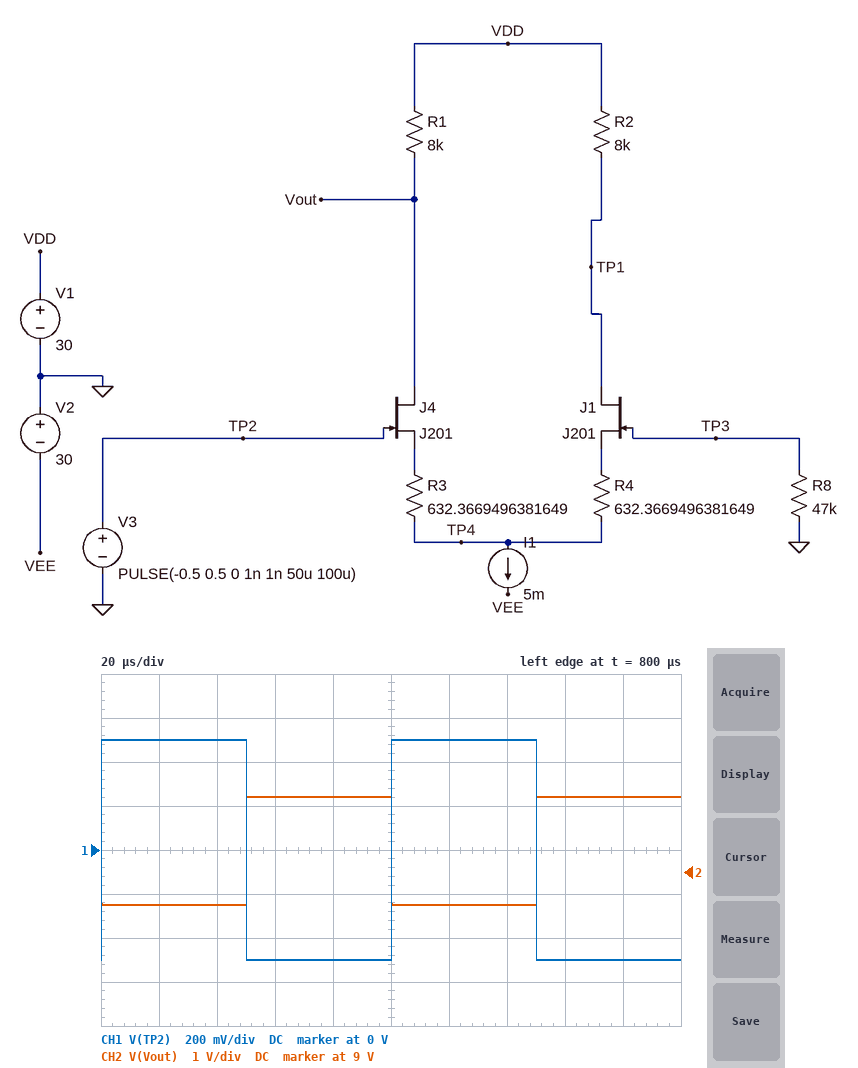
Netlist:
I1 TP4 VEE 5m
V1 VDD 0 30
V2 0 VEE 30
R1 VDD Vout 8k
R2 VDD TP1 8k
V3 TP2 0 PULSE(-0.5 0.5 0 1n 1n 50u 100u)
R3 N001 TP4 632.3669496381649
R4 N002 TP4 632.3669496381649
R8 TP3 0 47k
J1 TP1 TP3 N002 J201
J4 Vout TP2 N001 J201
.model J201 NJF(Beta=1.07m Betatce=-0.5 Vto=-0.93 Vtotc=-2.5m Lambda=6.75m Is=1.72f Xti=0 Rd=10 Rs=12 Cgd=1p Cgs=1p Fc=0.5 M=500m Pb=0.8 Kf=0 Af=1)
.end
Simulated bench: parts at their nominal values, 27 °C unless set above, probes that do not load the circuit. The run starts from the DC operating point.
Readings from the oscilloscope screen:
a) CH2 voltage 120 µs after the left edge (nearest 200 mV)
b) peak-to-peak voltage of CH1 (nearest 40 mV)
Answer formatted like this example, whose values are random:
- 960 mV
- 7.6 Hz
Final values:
- 8.2 V
- 1.00 V
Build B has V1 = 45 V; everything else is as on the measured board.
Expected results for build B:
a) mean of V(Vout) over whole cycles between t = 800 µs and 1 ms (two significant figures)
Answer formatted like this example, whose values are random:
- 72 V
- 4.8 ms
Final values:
- 25 V
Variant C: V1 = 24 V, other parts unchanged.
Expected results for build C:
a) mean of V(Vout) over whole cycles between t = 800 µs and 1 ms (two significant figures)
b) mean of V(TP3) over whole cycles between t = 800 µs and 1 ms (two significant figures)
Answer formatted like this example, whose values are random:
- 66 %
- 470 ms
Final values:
- 3.4 V
- -230 mV
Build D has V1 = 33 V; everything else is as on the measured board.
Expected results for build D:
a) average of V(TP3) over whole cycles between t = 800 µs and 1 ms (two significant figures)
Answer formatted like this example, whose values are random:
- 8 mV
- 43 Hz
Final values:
- -140 mV
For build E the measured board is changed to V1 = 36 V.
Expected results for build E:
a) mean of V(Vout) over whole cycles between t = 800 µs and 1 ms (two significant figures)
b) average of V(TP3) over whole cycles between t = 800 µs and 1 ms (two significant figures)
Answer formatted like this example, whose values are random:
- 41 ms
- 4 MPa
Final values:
- 16 V
- -110 mV
